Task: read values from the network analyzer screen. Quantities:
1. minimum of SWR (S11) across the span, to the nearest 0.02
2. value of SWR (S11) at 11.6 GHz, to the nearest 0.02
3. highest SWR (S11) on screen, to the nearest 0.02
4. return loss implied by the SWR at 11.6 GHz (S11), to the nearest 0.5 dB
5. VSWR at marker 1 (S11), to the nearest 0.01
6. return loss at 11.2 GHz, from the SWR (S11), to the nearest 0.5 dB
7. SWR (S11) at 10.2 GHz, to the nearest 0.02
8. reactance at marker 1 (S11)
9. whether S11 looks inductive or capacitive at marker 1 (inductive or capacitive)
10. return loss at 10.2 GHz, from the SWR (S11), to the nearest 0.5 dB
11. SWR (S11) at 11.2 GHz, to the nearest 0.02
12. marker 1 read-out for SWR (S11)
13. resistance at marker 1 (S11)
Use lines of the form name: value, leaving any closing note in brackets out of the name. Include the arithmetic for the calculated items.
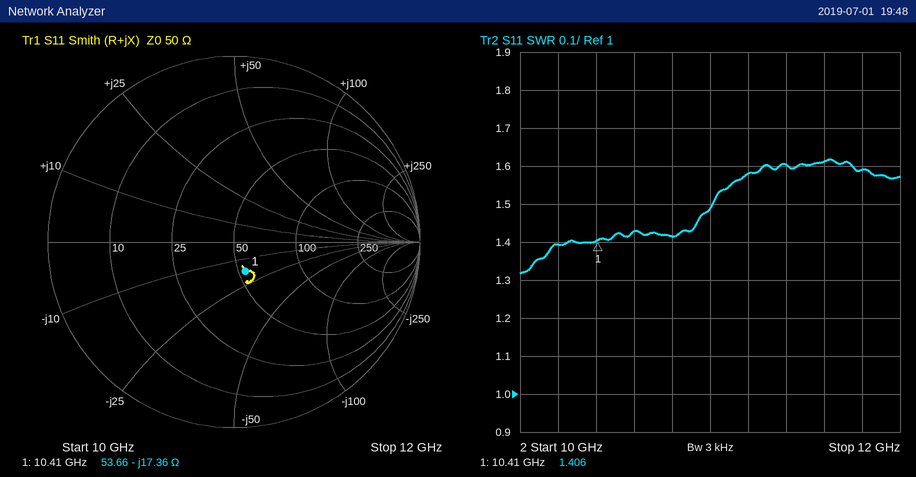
minimum of SWR (S11) across the span, to the nearest 0.02: 1.32
value of SWR (S11) at 11.6 GHz, to the nearest 0.02: 1.62
highest SWR (S11) on screen, to the nearest 0.02: 1.62
return loss implied by the SWR at 11.6 GHz (S11), to the nearest 0.5 dB: −20 log10((1.62 − 1)/(1.62 + 1)) ≈ 12.5 dB
VSWR at marker 1 (S11), to the nearest 0.01: 1.41
return loss at 11.2 GHz, from the SWR (S11), to the nearest 0.5 dB: −20 log10((1.58 − 1)/(1.58 + 1)) ≈ 13.0 dB
SWR (S11) at 10.2 GHz, to the nearest 0.02: 1.40
reactance at marker 1: -17.36 Ω
whether S11 looks inductive or capacitive at marker 1: capacitive
return loss at 10.2 GHz, from the SWR (S11), to the nearest 0.5 dB: −20 log10((1.4 − 1)/(1.4 + 1)) ≈ 15.6 dB, so 15.5 dB to the nearest 0.5 dB
SWR (S11) at 11.2 GHz, to the nearest 0.02: 1.58
marker 1 read-out for SWR: 1.406
resistance at marker 1: 53.66 Ω
